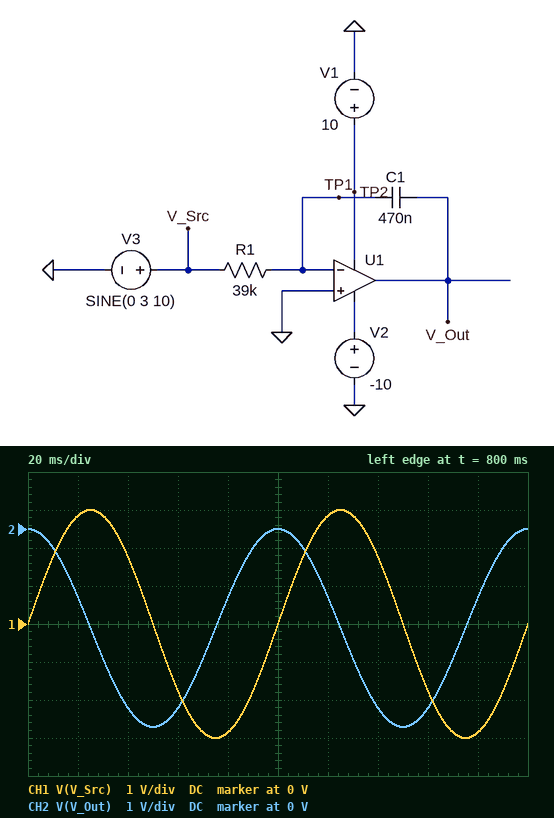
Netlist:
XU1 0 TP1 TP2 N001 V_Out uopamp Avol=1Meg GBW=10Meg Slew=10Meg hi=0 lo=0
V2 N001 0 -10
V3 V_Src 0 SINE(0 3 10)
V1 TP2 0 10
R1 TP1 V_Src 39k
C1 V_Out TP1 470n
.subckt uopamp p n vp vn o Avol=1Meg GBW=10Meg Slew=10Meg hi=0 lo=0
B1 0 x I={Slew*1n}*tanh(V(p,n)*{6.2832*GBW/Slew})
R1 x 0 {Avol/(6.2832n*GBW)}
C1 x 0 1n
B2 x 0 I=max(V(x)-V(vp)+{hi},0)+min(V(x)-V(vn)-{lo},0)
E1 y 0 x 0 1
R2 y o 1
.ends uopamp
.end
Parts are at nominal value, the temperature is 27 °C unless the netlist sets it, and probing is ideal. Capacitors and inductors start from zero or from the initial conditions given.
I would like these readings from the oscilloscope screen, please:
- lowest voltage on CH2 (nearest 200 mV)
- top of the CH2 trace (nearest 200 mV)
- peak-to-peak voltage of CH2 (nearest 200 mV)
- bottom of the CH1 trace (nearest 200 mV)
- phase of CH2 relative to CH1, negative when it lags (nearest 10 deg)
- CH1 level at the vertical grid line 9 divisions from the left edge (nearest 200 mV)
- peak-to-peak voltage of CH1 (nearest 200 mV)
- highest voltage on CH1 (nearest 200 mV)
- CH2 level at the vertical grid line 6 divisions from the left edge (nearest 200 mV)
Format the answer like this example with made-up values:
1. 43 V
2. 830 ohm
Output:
1. -5.2 V
2. 0 V
3. 5.2 V
4. -3.0 V
5. 90 deg
6. -2.8 V
7. 6.0 V
8. 3.0 V
9. -1.8 V
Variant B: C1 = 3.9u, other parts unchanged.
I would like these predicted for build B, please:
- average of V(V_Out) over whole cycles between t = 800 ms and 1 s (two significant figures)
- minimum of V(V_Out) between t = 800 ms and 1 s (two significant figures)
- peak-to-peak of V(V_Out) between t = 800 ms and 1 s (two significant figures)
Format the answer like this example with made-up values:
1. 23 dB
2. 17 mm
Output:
1. -310 mV
2. -630 mV
3. 630 mV
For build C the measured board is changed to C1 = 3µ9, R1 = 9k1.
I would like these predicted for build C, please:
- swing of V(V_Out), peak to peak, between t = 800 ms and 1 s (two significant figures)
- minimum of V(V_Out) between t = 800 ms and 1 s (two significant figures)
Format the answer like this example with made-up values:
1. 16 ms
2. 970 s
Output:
1. 2.7 V
2. -2.7 V
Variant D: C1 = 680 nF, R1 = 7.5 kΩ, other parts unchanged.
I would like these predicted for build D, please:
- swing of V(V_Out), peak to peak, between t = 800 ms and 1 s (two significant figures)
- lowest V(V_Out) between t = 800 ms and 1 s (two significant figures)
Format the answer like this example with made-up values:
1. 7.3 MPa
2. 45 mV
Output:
1. 19 V
2. -10 V
